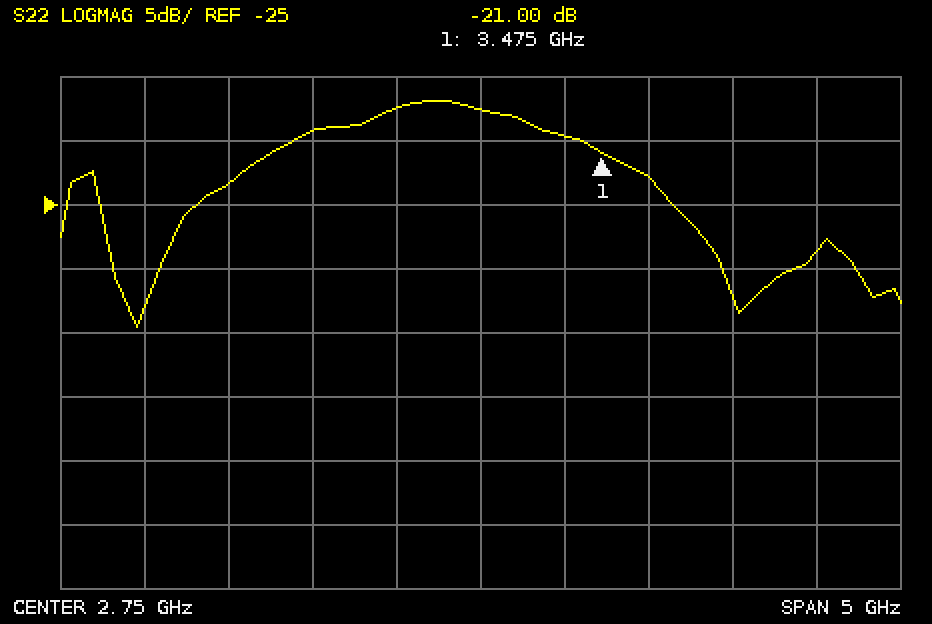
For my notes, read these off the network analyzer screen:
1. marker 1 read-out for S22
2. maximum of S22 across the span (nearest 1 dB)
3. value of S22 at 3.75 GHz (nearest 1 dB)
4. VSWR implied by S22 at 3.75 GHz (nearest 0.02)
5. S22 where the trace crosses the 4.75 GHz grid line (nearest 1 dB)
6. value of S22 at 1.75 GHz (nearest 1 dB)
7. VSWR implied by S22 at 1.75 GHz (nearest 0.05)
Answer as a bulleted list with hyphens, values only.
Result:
- -21.00 dB
- -17 dB
- -23 dB
- 1.16
- -29 dB
- -19 dB
- 1.25
